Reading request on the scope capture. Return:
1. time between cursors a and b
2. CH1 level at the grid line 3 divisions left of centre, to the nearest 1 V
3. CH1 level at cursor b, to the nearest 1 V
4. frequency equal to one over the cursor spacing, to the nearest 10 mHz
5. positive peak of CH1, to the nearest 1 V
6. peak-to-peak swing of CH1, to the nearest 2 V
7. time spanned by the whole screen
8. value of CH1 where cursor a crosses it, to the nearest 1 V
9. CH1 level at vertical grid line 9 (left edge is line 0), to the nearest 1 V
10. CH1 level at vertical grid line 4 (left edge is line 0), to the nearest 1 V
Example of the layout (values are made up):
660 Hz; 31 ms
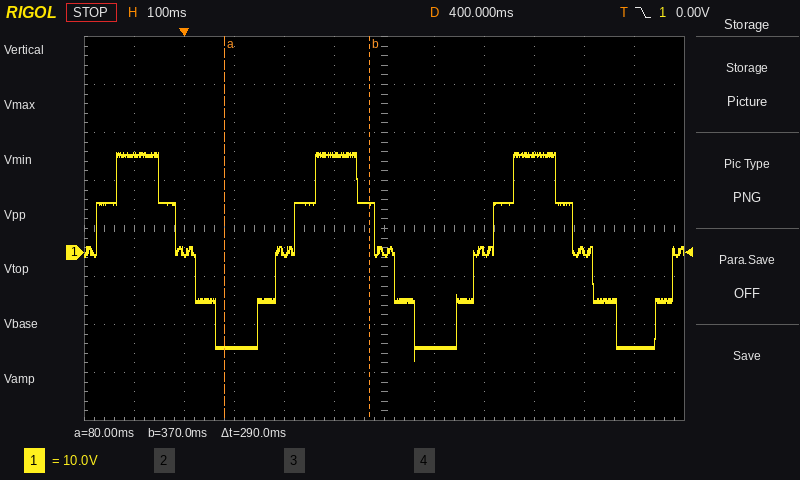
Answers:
290 ms; -20 V; 10 V; 3.45 Hz; 21 V; 44 V; 1.2 s; -20 V; 20 V; 0 V
